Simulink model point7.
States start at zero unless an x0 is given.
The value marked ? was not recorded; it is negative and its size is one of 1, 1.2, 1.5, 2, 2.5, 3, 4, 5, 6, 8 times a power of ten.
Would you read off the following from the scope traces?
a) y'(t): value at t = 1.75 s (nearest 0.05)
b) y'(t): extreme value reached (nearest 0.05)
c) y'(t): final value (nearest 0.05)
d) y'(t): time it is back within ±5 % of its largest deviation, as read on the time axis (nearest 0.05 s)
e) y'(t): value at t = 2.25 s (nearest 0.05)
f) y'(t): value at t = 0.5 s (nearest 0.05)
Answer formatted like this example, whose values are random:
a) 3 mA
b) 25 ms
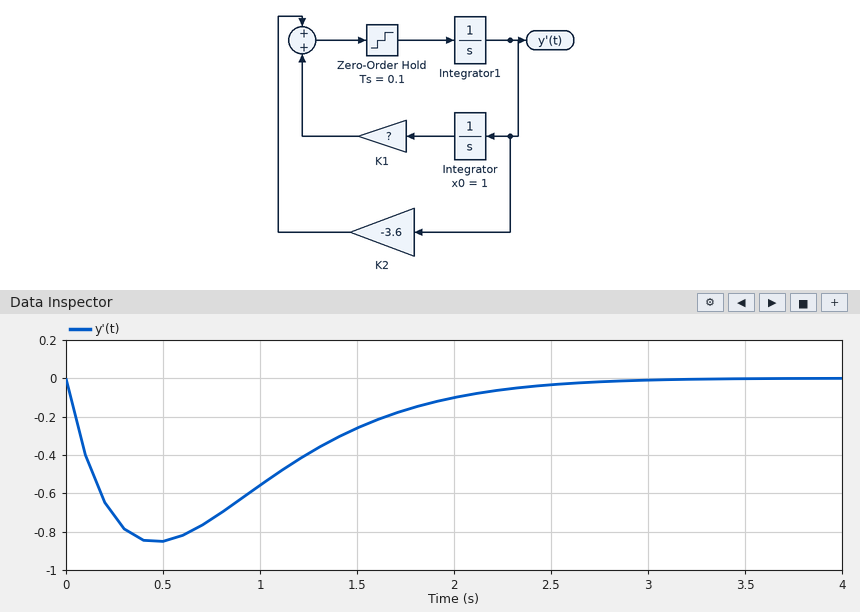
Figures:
a) -0.15
b) -0.85
c) 0.00
d) 2.40 s
e) -0.05
f) -0.85
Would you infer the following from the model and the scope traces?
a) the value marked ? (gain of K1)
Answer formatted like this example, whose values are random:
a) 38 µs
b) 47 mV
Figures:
a) -4
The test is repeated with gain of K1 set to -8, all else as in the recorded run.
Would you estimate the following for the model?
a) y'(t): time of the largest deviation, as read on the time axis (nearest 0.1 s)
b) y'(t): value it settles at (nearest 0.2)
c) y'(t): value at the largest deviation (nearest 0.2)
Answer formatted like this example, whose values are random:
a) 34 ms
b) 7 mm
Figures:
a) 0.4 s
b) 0.0
c) -1.6
